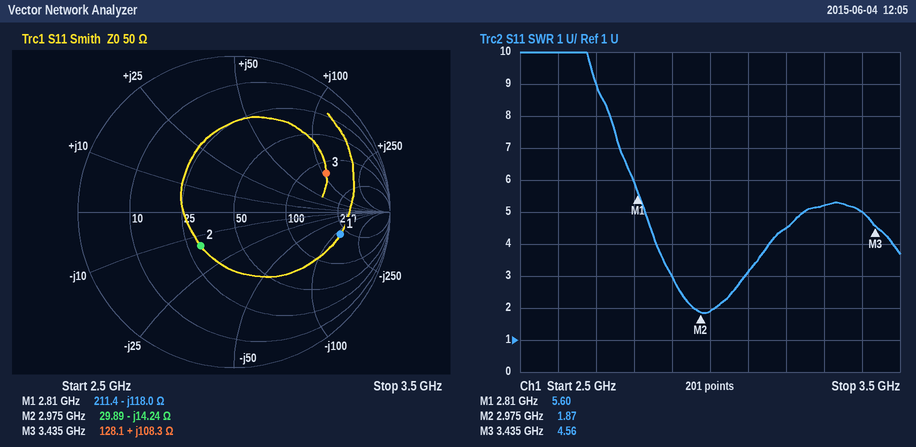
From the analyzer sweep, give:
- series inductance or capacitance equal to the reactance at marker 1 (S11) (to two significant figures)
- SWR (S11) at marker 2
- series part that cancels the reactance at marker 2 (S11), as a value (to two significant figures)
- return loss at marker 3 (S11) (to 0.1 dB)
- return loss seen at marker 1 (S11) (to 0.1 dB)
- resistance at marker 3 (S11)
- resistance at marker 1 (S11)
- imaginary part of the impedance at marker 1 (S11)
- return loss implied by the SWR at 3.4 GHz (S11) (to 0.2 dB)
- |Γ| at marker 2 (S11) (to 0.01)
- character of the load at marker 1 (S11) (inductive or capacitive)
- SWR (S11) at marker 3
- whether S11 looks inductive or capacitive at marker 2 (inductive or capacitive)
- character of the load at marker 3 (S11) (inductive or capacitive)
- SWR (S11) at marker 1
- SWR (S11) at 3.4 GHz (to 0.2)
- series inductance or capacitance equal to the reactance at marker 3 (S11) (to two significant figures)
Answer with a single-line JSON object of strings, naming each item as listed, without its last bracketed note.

{"series inductance or capacitance equal to the reactance at marker 1 (S11)": "480 fF", "SWR (S11) at marker 2": "1.87", "series part that cancels the reactance at marker 2 (S11), as a value": "760 pH", "return loss at marker 3 (S11)": "3.9 dB", "return loss seen at marker 1 (S11)": "3.1 dB", "resistance at marker 3": "128.1 Ω", "resistance at marker 1": "211.4 Ω", "imaginary part of the impedance at marker 1": "-118.0 Ω", "return loss implied by the SWR at 3.4 GHz (S11)": "3.6 dB", "|Γ| at marker 2 (S11)": "0.30", "character of the load at marker 1 (S11)": "capacitive", "SWR (S11) at marker 3": "4.56", "whether S11 looks inductive or capacitive at marker 2": "capacitive", "character of the load at marker 3 (S11)": "inductive", "SWR (S11) at marker 1": "5.60", "SWR (S11) at 3.4 GHz": "5.0", "series inductance or capacitance equal to the reactance at marker 3 (S11)": "5.0 nH"}
